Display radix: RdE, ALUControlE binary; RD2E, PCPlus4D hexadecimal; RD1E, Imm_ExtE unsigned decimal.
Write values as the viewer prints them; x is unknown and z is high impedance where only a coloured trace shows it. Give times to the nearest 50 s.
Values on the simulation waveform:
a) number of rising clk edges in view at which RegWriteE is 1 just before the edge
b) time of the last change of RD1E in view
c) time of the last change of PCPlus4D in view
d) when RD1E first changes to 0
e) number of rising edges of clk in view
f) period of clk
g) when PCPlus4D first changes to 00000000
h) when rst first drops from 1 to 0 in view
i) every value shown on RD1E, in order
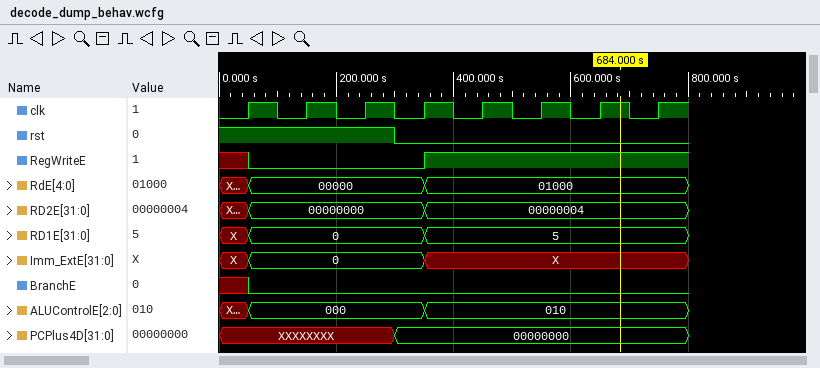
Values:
4
350 s
300 s
50 s
8
100 s
300 s
300 s
X, 0, 5
